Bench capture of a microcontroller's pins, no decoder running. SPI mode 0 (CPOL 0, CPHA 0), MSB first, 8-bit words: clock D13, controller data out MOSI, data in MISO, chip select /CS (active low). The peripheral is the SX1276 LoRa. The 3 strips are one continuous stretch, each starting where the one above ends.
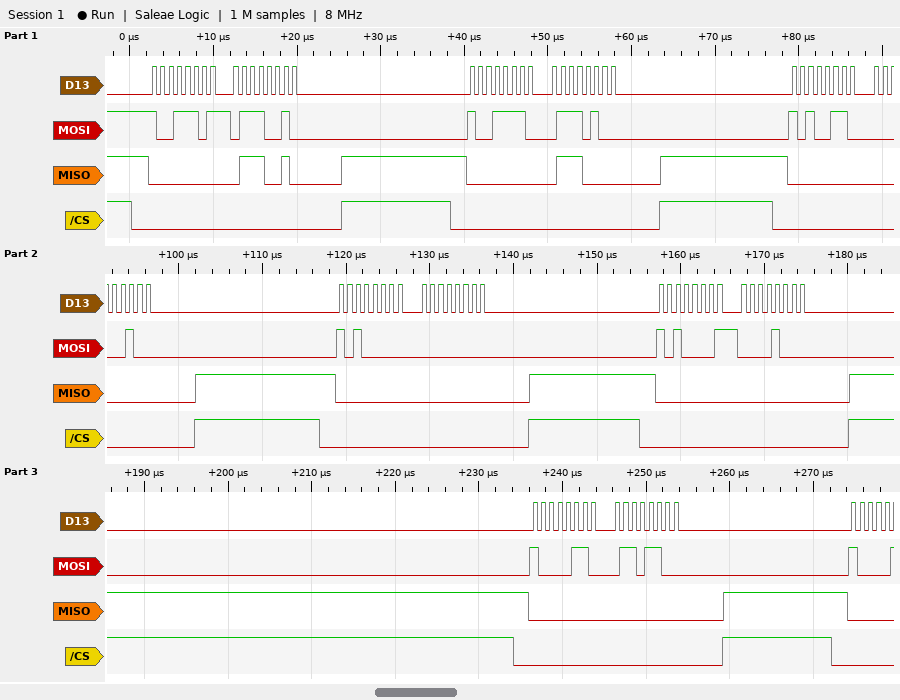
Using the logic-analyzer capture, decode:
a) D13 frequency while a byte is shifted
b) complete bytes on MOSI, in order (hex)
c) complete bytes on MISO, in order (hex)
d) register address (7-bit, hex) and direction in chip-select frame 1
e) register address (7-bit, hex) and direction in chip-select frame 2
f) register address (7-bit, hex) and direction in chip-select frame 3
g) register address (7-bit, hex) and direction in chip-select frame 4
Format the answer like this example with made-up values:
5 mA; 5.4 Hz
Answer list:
1 MHz; 9D 72 9E 74 A6 04 A0 00 A1 08 86 6C; 00 72 00 70 00 00 00 00 00 00 00 00; 0x1D write; 0x1E write; 0x26 write; 0x20 write
